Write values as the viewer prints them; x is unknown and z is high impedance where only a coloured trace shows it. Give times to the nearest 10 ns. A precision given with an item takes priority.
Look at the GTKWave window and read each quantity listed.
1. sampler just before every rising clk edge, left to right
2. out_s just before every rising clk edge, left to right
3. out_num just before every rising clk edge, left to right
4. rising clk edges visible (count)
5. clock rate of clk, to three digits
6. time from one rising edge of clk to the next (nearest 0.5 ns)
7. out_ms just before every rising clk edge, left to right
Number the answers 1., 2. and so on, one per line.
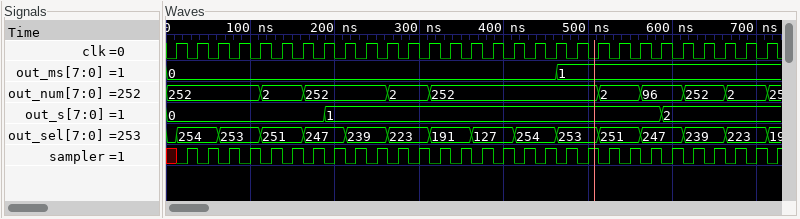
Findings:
1. x 1 1 1 1 1 1 1 1 1 1 1 1 1 1 1 1 1 1 1 1 1 1 1 1 1 1 1 1
2. 0, 0, 0, 0, 0, 0, 0, 0, 1, 1, 1, 1, 1, 1, 1, 1, 1, 1, 1, 1, 1, 1, 1, 1, 2, 2, 2, 2, 2
3. 252, 252, 252, 252, 252, 2, 2, 252, 252, 252, 252, 2, 2, 252, 252, 252, 252, 252, 252, 252, 252, 2, 2, 96, 96, 252, 252, 2, 2
4. 29
5. 40.0 MHz
6. 25 ns
7. 0, 0, 0, 0, 0, 0, 0, 0, 0, 0, 0, 0, 0, 0, 0, 0, 0, 0, 0, 1, 1, 1, 1, 1, 1, 1, 1, 1, 1
